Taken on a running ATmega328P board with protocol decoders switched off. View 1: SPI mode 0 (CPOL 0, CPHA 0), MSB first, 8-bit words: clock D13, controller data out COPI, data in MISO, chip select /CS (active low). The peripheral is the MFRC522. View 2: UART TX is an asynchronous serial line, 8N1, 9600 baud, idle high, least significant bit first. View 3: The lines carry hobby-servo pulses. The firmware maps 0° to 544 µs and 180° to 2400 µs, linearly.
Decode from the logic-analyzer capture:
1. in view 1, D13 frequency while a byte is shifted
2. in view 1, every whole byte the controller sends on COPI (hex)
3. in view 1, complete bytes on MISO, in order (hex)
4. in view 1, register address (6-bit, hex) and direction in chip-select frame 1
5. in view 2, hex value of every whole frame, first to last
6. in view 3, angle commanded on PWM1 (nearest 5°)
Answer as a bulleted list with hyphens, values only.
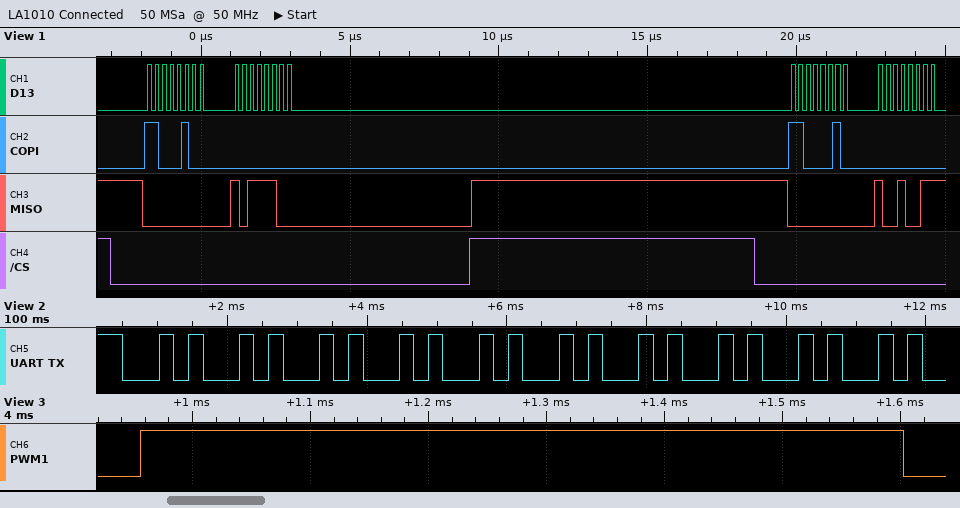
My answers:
- 4 MHz
- 0xC4 0x00 0xC2 0x00
- 0x00 0xBC 0x00 0x93
- 0x22 read
- 30 30 30 30 30 30 30 30 30 30
- 10°
